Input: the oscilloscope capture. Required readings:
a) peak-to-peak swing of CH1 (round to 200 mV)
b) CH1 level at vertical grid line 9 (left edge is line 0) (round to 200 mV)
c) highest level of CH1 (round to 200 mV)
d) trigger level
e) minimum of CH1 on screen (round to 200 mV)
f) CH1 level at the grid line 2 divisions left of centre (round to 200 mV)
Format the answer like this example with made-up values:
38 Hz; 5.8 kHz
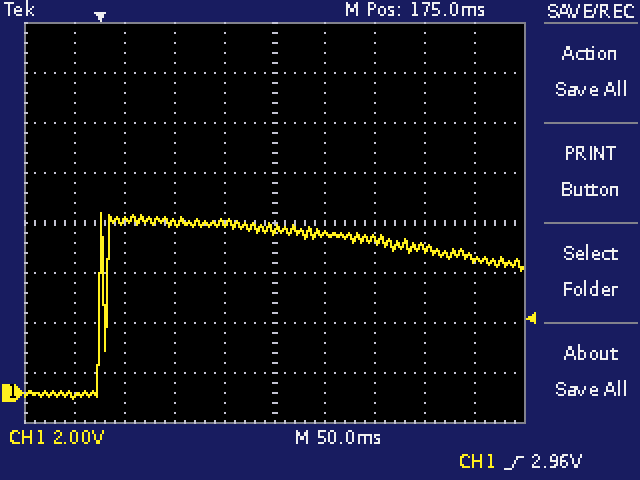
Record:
7.4 V; 5.4 V; 7.2 V; 2.96 V; -200 mV; 6.8 V
